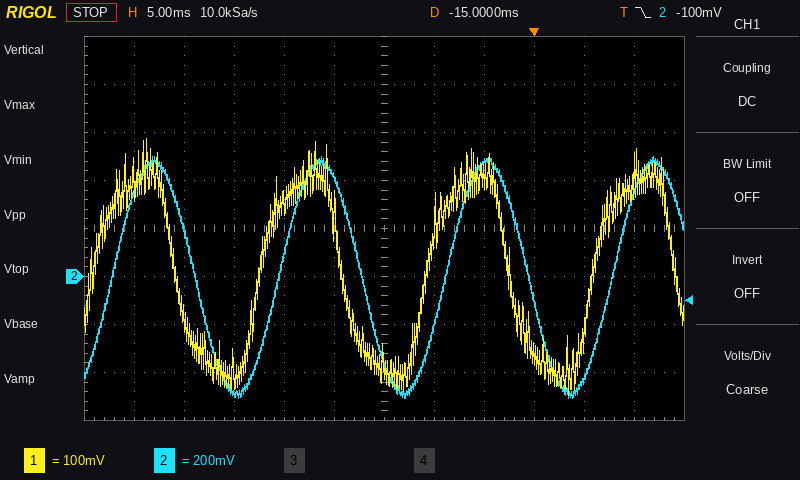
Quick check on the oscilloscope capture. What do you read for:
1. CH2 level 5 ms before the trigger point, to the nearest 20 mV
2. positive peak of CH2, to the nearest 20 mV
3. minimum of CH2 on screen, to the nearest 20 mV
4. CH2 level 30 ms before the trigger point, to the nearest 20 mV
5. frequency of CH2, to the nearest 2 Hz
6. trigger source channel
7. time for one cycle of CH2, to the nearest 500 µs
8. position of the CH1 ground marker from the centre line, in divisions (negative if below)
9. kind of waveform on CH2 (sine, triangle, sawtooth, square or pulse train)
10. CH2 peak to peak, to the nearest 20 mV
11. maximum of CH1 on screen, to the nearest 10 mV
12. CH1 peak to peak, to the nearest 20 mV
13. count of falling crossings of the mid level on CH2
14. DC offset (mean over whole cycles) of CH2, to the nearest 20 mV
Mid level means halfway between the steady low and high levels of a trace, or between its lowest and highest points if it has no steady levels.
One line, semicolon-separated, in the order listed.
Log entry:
480 mV; 500 mV; -500 mV; -480 mV; 60 Hz; CH2; 16.5 ms; -1.0 div; sine; 1.00 V; 290 mV; 540 mV; 3; 0 mV
